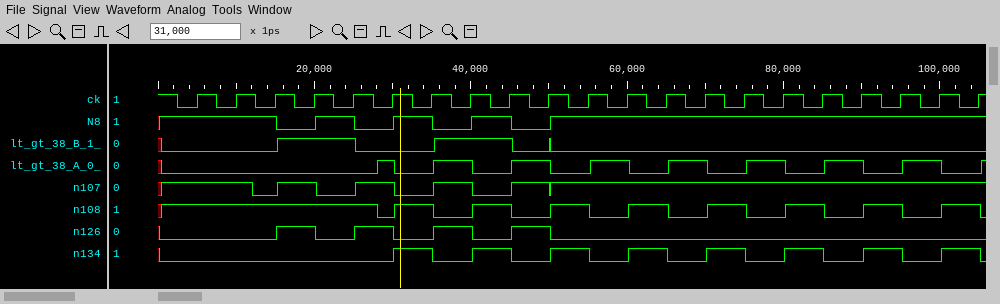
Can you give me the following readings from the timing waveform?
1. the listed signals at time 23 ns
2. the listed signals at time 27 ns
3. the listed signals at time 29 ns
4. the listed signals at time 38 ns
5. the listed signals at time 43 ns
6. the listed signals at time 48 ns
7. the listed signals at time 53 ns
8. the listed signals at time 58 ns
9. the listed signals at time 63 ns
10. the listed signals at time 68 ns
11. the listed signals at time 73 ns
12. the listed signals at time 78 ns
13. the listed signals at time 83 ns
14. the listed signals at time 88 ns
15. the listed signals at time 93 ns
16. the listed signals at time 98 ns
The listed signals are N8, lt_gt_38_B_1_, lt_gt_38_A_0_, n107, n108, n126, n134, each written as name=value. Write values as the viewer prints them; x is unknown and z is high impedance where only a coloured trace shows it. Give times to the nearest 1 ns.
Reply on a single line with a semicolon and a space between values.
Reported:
N8=1, lt_gt_38_B_1_=1, lt_gt_38_A_0_=0, n107=0, n108=1, n126=0, n134=0; N8=0, lt_gt_38_B_1_=0, lt_gt_38_A_0_=0, n107=1, n108=1, n126=1, n134=0; N8=0, lt_gt_38_B_1_=0, lt_gt_38_A_0_=1, n107=1, n108=0, n126=1, n134=0; N8=0, lt_gt_38_B_1_=1, lt_gt_38_A_0_=1, n107=1, n108=0, n126=1, n134=0; N8=1, lt_gt_38_B_1_=1, lt_gt_38_A_0_=0, n107=0, n108=1, n126=0, n134=1; N8=0, lt_gt_38_B_1_=0, lt_gt_38_A_0_=1, n107=1, n108=0, n126=1, n134=0; N8=1, lt_gt_38_B_1_=0, lt_gt_38_A_0_=0, n107=1, n108=1, n126=0, n134=1; N8=1, lt_gt_38_B_1_=0, lt_gt_38_A_0_=1, n107=1, n108=0, n126=0, n134=0; N8=1, lt_gt_38_B_1_=0, lt_gt_38_A_0_=0, n107=1, n108=1, n126=0, n134=1; N8=1, lt_gt_38_B_1_=0, lt_gt_38_A_0_=1, n107=1, n108=0, n126=0, n134=0; N8=1, lt_gt_38_B_1_=0, lt_gt_38_A_0_=0, n107=1, n108=1, n126=0, n134=1; N8=1, lt_gt_38_B_1_=0, lt_gt_38_A_0_=1, n107=1, n108=0, n126=0, n134=0; N8=1, lt_gt_38_B_1_=0, lt_gt_38_A_0_=0, n107=1, n108=1, n126=0, n134=1; N8=1, lt_gt_38_B_1_=0, lt_gt_38_A_0_=1, n107=1, n108=0, n126=0, n134=0; N8=1, lt_gt_38_B_1_=0, lt_gt_38_A_0_=0, n107=1, n108=1, n126=0, n134=1; N8=1, lt_gt_38_B_1_=0, lt_gt_38_A_0_=1, n107=1, n108=0, n126=0, n134=0
